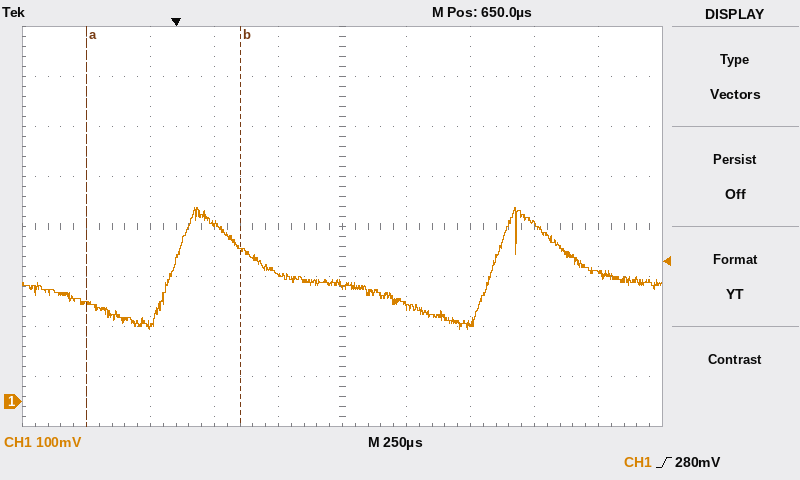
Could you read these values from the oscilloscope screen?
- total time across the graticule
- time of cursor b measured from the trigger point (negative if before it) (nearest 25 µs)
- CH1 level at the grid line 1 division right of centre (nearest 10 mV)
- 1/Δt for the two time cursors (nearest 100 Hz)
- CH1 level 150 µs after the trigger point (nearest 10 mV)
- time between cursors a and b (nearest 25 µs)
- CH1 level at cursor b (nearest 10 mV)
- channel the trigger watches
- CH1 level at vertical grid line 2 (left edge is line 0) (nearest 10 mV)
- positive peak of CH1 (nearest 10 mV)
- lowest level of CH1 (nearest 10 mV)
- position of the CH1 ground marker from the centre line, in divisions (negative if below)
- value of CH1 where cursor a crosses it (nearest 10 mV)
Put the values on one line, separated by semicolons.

2.5 ms; +250 µs; 190 mV; 1.7 kHz; 360 mV; 600 µs; 310 mV; CH1; 150 mV; 390 mV; 140 mV; -3.5 div; 200 mV
